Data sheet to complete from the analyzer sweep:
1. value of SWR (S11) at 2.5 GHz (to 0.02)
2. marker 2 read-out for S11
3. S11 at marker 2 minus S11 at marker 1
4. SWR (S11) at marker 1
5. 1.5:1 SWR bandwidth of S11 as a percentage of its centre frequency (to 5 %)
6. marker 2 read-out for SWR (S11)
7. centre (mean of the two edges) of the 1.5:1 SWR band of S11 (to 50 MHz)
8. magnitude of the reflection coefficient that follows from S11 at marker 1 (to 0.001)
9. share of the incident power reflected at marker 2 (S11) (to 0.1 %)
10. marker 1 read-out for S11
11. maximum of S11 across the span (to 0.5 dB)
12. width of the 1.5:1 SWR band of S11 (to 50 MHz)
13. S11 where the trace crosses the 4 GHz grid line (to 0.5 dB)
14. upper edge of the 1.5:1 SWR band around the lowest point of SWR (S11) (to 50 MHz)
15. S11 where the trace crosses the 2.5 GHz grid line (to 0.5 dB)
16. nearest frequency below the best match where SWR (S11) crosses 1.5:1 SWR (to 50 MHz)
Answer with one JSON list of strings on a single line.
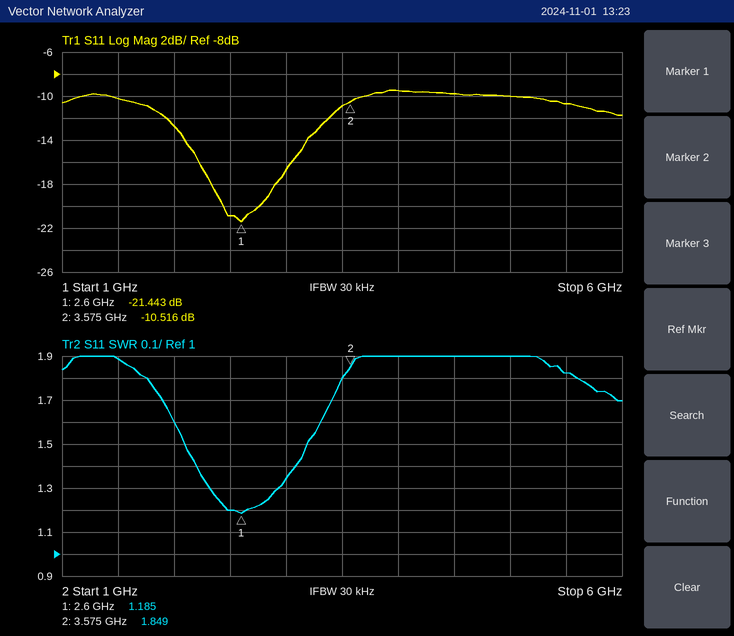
["1.20", "-10.516 dB", "10.927 dB", "1.185", "40 %", "1.849", "2.65 GHz", "0.085", "8.9 %", "-21.443 dB", "-9.5 dB", "1.10 GHz", "-9.5 dB", "3.20 GHz", "-21.0 dB", "2.10 GHz"]
